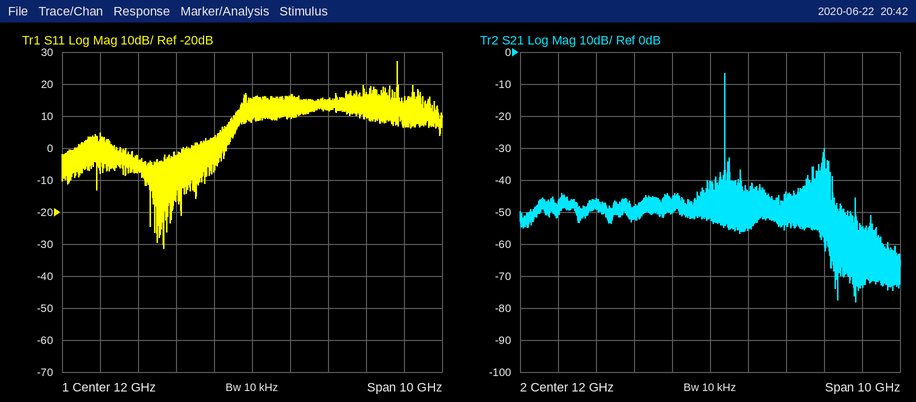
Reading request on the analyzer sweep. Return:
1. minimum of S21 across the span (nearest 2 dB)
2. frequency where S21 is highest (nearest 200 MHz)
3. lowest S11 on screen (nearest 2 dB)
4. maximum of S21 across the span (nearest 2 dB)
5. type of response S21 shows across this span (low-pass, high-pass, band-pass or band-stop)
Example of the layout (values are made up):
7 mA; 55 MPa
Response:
-78 dB; 12.4 GHz; -32 dB; -6 dB; band-pass
